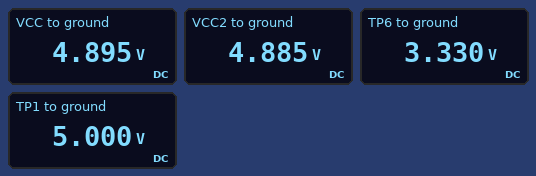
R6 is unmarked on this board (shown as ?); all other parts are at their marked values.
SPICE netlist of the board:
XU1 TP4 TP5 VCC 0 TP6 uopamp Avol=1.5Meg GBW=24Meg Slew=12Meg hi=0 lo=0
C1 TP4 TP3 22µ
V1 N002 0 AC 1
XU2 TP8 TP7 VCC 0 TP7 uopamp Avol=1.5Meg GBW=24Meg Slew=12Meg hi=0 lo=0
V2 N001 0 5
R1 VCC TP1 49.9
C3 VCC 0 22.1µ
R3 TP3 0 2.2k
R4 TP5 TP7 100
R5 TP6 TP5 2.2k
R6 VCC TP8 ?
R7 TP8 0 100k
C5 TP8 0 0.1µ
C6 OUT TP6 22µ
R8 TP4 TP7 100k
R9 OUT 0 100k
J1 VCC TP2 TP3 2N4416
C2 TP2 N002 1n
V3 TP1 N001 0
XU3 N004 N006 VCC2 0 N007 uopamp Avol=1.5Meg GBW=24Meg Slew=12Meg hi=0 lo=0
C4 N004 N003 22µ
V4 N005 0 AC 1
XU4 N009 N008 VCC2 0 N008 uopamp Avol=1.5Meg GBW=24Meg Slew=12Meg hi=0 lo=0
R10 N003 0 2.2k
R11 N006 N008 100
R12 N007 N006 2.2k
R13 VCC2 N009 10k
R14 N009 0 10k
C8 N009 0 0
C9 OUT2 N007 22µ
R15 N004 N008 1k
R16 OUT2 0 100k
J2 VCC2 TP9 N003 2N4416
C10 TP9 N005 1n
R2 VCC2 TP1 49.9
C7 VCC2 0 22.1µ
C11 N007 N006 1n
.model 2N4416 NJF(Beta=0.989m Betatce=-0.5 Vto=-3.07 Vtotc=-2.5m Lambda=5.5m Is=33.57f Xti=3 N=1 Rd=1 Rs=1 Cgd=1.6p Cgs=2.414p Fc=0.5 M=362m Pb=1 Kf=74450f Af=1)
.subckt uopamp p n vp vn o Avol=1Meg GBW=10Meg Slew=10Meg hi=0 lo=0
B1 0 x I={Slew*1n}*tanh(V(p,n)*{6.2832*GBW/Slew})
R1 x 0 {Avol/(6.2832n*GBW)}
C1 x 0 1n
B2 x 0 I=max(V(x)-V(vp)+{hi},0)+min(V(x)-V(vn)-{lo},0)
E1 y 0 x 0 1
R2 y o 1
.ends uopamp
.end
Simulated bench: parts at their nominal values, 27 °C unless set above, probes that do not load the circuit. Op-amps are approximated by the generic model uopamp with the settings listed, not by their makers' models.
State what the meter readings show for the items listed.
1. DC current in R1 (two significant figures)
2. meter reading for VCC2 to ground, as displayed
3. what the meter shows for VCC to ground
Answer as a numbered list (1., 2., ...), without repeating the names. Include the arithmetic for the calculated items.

1. (5 V - 4.895 V) / 49.9 Ω = 2.1 mA
2. 4.885 V
3. 4.895 V
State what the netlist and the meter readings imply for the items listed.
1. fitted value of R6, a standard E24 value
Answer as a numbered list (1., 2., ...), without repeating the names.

1. 47 kΩ
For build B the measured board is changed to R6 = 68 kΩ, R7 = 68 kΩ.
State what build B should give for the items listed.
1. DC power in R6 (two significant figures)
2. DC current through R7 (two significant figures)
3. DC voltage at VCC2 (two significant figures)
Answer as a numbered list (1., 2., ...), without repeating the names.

1. 88 µW
2. 36 µA
3. 4.9 V
